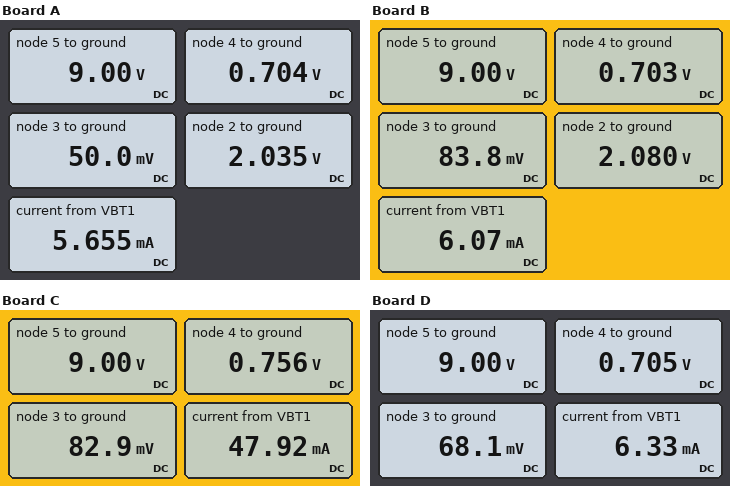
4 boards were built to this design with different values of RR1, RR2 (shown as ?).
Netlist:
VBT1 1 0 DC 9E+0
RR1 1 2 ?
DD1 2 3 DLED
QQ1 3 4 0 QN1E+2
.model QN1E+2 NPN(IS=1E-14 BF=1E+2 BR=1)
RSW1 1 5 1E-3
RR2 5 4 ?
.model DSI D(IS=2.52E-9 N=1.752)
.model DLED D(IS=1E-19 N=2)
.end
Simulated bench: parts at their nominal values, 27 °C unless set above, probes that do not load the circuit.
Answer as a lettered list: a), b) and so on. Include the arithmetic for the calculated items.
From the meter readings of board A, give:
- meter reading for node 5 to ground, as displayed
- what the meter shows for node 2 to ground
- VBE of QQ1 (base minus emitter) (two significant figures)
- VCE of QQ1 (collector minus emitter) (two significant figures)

a) 9.00 V
b) 2.035 V
c) 704 mV = 700 mV
d) 50 mV = 50 mV
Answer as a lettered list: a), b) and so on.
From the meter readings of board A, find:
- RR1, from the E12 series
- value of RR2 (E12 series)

a) 1.5 kΩ
b) 8.2 kΩ
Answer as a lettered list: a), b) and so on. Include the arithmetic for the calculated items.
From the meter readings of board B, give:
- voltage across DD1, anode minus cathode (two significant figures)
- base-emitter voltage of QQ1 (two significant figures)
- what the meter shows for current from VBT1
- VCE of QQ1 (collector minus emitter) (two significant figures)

a) 2.08 V - 83.8 mV = 2.0 V
b) 703 mV = 700 mV
c) 6.07 mA
d) 83.8 mV = 84 mV
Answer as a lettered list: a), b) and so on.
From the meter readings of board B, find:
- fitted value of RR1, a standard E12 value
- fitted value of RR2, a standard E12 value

a) 1.2 kΩ
b) 27 kΩ
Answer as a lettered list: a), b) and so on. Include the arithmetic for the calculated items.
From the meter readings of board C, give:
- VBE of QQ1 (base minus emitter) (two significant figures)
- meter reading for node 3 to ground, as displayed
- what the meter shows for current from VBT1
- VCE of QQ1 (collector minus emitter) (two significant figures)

a) 756 mV = 760 mV
b) 82.9 mV
c) 47.92 mA
d) 82.9 mV = 83 mV
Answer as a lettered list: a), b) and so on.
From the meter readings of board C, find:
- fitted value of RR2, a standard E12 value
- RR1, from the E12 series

a) 3.3 kΩ
b) 150 Ω
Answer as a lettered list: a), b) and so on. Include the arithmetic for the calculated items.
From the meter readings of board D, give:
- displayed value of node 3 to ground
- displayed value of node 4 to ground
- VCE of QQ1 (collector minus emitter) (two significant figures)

a) 68.1 mV
b) 0.705 V
c) 68.1 mV = 68 mV
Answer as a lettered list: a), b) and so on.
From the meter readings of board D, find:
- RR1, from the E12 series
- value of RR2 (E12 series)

a) 1.2 kΩ
b) 15 kΩ
